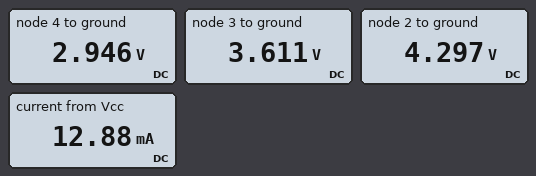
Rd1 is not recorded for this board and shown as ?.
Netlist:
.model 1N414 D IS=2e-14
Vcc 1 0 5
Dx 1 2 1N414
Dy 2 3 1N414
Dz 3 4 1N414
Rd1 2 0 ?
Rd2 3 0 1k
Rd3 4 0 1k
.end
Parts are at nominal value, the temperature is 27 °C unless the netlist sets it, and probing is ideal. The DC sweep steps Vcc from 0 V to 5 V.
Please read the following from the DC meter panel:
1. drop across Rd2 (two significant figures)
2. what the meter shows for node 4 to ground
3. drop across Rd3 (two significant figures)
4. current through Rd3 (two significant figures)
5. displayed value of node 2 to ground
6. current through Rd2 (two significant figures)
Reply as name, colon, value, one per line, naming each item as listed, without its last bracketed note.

drop across Rd2: 3.6 V
what the meter shows for node 4 to ground: 2.946 V
drop across Rd3: 2.9 V
current through Rd3: 2.9 mA
displayed value of node 2 to ground: 4.297 V
current through Rd2: 3.6 mA
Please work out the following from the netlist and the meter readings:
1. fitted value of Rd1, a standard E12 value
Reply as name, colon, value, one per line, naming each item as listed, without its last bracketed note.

fitted value of Rd1, a standard E12 value: 680 Ω
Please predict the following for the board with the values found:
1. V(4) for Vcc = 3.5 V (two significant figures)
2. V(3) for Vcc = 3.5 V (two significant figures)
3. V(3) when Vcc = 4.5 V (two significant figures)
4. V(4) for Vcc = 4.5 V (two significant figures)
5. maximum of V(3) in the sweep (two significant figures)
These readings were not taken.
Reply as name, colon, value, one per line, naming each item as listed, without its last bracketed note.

V(4) for Vcc = 3.5 V: 1.5 V
V(3) for Vcc = 3.5 V: 2.1 V
V(3) when Vcc = 4.5 V: 3.1 V
V(4) for Vcc = 4.5 V: 2.5 V
maximum of V(3) in the sweep: 3.6 V
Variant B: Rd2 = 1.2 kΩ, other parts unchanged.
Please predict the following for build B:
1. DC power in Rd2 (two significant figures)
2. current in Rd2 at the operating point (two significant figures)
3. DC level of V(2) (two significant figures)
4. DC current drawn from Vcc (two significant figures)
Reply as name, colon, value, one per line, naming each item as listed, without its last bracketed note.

DC power in Rd2: 11 mW
current in Rd2 at the operating point: 3.0 mA
DC level of V(2): 4.3 V
DC current drawn from Vcc: 12 mA
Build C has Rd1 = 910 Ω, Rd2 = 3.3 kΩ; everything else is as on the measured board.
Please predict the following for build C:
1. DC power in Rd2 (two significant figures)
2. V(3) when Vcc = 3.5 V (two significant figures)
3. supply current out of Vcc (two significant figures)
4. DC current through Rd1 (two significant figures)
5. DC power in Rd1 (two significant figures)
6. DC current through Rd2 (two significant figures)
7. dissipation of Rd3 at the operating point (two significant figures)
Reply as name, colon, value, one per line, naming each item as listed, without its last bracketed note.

DC power in Rd2: 4.0 mW
V(3) when Vcc = 3.5 V: 2.2 V
supply current out of Vcc: 8.8 mA
DC current through Rd1: 4.7 mA
DC power in Rd1: 20 mW
DC current through Rd2: 1.1 mA
dissipation of Rd3 at the operating point: 8.8 mW
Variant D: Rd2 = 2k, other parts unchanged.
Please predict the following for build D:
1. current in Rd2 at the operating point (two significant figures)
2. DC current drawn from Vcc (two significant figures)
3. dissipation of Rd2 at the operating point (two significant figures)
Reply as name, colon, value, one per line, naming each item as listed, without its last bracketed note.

current in Rd2 at the operating point: 1.8 mA
DC current drawn from Vcc: 11 mA
dissipation of Rd2 at the operating point: 6.6 mW
